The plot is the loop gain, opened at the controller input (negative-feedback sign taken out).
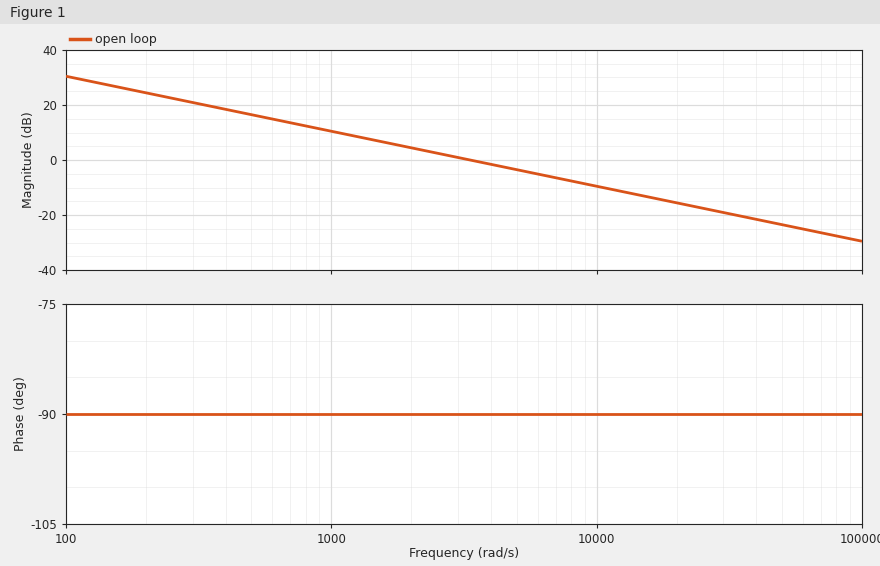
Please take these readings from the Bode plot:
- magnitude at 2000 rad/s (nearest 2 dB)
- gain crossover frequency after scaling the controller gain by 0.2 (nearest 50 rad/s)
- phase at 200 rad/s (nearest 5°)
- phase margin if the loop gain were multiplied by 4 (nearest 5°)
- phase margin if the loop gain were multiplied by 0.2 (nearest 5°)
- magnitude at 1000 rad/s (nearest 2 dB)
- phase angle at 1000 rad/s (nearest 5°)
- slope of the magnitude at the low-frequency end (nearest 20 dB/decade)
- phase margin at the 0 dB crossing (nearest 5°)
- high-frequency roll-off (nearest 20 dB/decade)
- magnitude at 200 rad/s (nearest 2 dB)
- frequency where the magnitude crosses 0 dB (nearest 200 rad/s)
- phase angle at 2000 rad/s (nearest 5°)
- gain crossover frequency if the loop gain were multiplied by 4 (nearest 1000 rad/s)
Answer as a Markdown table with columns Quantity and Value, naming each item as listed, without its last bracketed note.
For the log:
| Quantity | Value |
|---|---|
| magnitude at 2000 rad/s | 4 dB |
| gain crossover frequency after scaling the controller gain by 0.2 | 650 rad/s |
| phase at 200 rad/s | -90° |
| phase margin if the loop gain were multiplied by 4 | 90° |
| phase margin if the loop gain were multiplied by 0.2 | 90° |
| magnitude at 1000 rad/s | 10 dB |
| phase angle at 1000 rad/s | -90° |
| slope of the magnitude at the low-frequency end | -20 dB/decade |
| phase margin at the 0 dB crossing | 90° |
| high-frequency roll-off | -20 dB/decade |
| magnitude at 200 rad/s | 24 dB |
| frequency where the magnitude crosses 0 dB | 3400 rad/s |
| phase angle at 2000 rad/s | -90° |
| gain crossover frequency if the loop gain were multiplied by 4 | 13000 rad/s |
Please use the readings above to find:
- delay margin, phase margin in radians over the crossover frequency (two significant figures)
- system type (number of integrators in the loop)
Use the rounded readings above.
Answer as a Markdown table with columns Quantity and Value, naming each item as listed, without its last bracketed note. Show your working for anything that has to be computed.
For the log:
| Quantity | Value |
|---|---|
| delay margin, phase margin in radians over the crossover frequency | 90 × π / 180 / 3400 = 0.00046 s |
| system type | 1 |
